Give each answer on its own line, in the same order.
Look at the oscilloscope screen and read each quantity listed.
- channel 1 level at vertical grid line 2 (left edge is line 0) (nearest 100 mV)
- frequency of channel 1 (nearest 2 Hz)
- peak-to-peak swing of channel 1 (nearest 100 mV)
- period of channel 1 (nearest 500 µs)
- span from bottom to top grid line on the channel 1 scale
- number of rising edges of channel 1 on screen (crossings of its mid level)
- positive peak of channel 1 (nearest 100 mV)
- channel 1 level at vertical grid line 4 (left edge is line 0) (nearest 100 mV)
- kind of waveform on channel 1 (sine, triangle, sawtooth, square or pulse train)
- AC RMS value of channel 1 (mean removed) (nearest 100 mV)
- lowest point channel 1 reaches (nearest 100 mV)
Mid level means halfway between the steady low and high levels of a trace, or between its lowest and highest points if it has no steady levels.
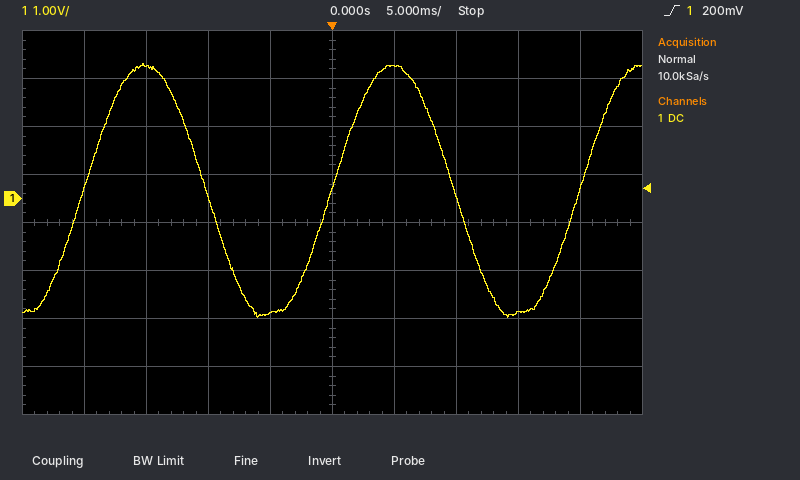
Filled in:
2.8 V
50 Hz
5.3 V
20.0 ms
8 V
3
2.8 V
-2.4 V
sine
1.9 V
-2.5 V
